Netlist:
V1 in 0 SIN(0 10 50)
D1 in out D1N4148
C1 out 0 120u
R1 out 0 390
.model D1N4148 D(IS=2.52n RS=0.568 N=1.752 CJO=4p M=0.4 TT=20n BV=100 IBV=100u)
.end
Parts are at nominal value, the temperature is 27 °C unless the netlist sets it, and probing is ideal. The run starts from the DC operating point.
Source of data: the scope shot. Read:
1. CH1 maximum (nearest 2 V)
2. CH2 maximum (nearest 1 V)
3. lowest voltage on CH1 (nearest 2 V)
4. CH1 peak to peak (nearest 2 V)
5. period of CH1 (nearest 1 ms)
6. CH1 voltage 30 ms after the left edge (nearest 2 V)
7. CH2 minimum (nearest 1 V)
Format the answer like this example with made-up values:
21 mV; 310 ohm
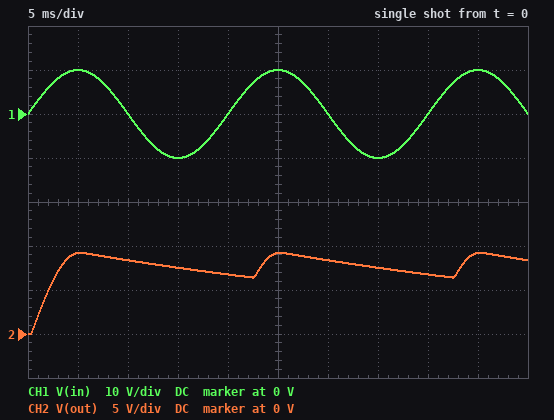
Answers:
10 V; 9 V; -10 V; 20 V; 20 ms; 0 V; 0 V
